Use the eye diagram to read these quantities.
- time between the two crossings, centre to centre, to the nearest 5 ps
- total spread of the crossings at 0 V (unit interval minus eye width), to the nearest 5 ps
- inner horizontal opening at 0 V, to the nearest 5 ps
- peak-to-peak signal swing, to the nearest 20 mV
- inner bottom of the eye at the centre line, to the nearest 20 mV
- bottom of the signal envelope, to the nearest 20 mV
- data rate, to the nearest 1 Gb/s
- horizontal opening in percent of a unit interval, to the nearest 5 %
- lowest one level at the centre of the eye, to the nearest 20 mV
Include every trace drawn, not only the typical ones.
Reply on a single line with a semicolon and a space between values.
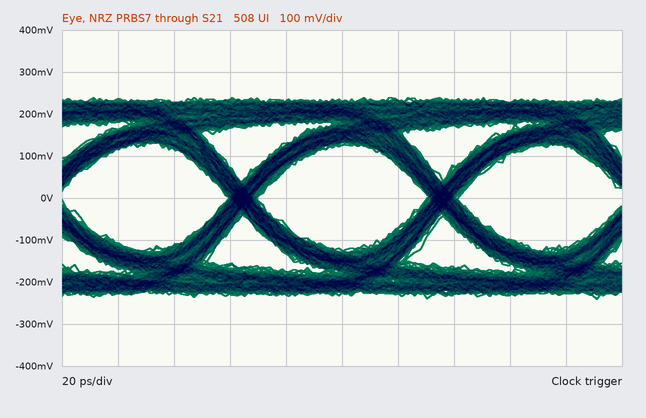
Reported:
70 ps; 10 ps; 60 ps; 480 mV; -120 mV; -240 mV; 14 Gb/s; 85 %; 120 mV
